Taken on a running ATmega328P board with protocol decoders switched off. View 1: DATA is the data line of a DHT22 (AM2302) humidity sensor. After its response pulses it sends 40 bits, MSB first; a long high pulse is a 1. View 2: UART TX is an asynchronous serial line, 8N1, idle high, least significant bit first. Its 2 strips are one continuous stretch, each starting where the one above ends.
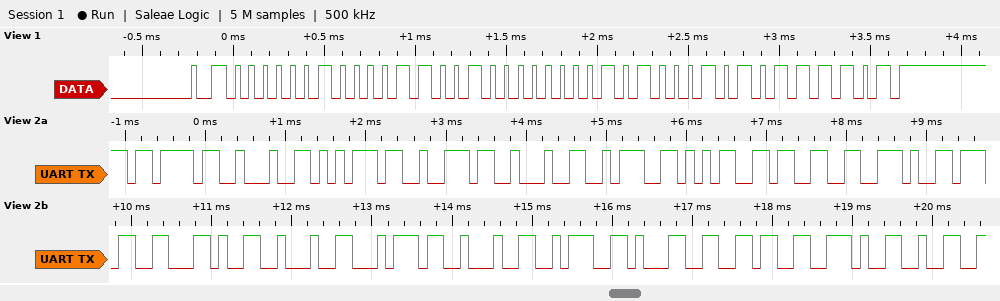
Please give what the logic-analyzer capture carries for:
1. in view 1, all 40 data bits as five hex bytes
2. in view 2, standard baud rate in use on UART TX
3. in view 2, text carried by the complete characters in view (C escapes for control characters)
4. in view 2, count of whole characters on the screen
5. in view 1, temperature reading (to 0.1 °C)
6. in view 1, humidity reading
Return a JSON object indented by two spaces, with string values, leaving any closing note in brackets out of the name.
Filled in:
{
  "in view 1, all 40 data bits as five hex bytes": "02 19 00 A2 BD",
  "in view 2, standard baud rate in use on UART TX": "9600 baud",
  "in view 2, text carried by the complete characters in view": "\"{\\\"ur\\\":53.7,\\\"t\\\":16.2\"",
  "in view 2, count of whole characters on the screen": "19",
  "in view 1, temperature reading": "16.2 °C",
  "in view 1, humidity reading": "53.7 %"
}
